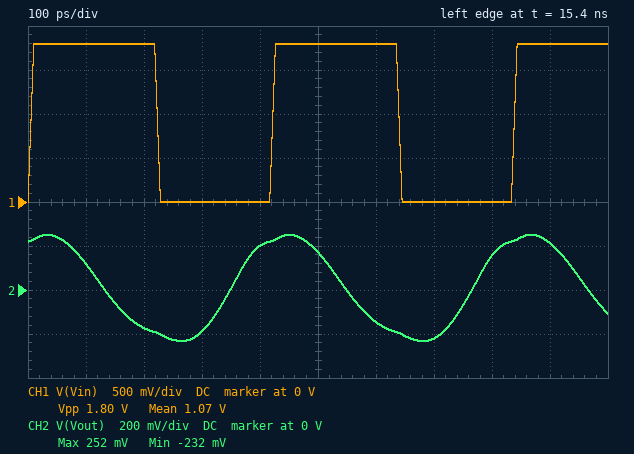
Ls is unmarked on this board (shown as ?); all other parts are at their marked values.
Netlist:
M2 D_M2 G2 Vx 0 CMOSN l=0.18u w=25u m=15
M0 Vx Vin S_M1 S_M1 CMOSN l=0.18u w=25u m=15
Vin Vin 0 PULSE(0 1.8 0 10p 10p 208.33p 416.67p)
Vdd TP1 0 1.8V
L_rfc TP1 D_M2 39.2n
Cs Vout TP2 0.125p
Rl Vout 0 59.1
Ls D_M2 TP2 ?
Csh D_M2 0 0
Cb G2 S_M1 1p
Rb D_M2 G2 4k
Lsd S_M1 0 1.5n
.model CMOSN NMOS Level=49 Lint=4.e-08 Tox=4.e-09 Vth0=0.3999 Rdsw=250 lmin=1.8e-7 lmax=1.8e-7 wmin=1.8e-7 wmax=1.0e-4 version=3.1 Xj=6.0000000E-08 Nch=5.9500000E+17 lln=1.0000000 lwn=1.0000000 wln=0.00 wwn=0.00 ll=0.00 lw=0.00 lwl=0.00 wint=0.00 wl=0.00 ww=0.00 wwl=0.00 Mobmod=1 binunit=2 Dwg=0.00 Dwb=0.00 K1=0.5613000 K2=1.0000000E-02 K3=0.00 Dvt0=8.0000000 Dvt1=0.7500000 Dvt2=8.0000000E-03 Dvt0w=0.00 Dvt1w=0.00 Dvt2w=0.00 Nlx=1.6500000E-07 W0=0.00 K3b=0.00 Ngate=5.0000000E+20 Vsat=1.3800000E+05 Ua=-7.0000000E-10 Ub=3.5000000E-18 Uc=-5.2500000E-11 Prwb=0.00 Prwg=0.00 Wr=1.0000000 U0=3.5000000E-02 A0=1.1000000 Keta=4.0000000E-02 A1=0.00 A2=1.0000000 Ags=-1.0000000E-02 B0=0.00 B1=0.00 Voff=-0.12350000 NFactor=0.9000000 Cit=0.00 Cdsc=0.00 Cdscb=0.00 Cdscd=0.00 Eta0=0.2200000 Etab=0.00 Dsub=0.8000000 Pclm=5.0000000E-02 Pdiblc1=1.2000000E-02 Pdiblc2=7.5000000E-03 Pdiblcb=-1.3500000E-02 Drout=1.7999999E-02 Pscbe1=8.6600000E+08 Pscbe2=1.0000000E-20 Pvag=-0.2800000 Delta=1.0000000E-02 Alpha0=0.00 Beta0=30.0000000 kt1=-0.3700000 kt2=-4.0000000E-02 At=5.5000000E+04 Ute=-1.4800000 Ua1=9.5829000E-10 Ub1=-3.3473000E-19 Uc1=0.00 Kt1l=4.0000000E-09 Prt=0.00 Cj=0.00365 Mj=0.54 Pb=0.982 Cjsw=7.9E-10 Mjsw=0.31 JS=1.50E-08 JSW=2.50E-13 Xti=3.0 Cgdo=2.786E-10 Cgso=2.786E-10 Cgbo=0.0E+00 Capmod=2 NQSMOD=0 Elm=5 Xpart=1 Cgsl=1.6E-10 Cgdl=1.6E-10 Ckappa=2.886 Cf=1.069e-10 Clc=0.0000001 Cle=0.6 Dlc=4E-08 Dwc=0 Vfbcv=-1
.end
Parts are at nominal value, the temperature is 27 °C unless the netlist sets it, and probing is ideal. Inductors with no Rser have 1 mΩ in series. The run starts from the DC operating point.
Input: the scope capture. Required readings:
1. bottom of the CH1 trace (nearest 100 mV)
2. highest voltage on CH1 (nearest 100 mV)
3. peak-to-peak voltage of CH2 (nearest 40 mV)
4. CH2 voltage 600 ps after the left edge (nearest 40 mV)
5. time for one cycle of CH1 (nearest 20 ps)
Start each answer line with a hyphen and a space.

- 0 V
- 1.8 V
- 480 mV
- -160 mV
- 420 ps
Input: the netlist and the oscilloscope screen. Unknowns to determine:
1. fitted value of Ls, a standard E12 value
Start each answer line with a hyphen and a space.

- 82 nH
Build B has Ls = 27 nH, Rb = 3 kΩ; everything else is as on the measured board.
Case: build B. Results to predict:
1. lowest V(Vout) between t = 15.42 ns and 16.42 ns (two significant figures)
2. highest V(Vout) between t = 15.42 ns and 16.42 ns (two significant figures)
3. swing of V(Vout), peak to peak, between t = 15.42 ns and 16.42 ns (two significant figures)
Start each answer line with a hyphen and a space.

- -1.6 V
- 1.4 V
- 3.0 V
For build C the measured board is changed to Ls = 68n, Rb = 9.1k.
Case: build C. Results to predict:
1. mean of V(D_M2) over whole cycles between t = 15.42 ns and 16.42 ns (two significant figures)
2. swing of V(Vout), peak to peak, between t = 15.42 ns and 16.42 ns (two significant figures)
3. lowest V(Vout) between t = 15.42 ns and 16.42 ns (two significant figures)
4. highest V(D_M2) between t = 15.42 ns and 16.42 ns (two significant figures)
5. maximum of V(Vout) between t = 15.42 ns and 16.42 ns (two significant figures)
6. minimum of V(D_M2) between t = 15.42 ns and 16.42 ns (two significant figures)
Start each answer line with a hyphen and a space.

- 1.8 V
- 670 mV
- -330 mV
- 6.8 V
- 340 mV
- -1.1 V
